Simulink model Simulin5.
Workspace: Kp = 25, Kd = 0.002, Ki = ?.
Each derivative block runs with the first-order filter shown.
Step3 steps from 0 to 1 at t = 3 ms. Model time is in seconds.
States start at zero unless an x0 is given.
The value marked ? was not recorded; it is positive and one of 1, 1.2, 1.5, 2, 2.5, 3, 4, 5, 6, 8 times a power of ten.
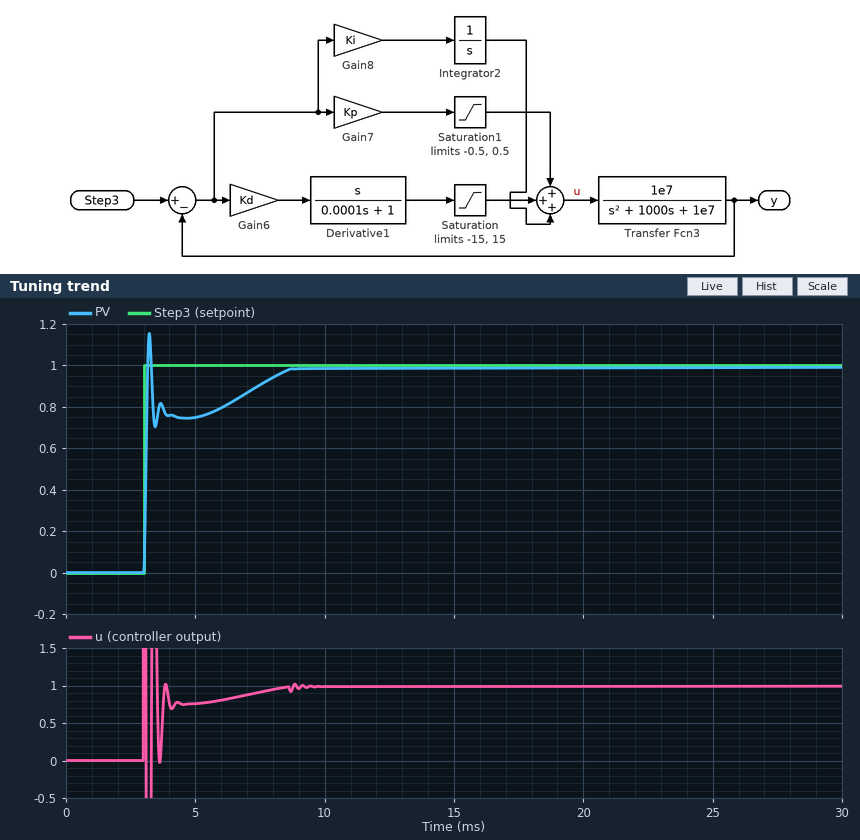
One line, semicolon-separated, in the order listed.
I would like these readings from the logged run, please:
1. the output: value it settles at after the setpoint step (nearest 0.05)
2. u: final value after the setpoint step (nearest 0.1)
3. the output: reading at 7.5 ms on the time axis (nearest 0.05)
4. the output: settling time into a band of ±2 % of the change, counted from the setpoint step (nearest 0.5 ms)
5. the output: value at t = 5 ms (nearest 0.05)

1.00; 1.0; 0.90; 5.5 ms; 0.75
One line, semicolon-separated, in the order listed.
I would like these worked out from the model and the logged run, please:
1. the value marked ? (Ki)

600
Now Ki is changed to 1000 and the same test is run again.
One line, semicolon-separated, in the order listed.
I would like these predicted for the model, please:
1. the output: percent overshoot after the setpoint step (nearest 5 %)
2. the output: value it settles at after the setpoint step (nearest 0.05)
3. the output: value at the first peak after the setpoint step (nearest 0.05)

15 %; 1.00; 1.15
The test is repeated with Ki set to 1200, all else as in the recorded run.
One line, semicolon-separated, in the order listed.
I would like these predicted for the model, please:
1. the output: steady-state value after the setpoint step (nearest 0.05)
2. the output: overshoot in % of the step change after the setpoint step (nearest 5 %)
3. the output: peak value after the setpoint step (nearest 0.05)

1.00; 15 %; 1.15
